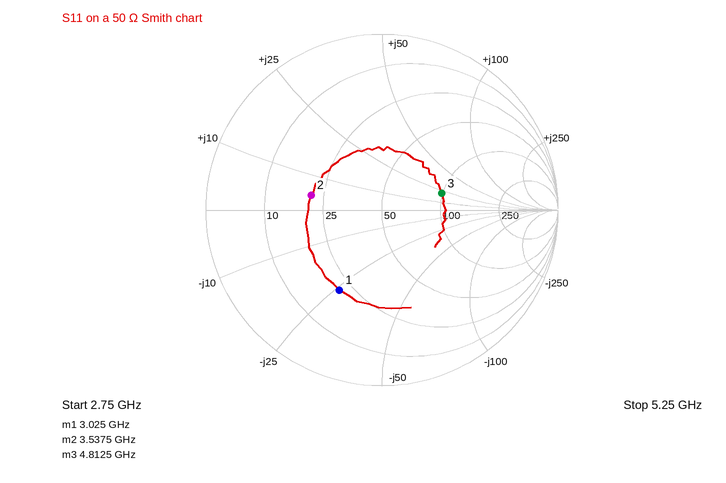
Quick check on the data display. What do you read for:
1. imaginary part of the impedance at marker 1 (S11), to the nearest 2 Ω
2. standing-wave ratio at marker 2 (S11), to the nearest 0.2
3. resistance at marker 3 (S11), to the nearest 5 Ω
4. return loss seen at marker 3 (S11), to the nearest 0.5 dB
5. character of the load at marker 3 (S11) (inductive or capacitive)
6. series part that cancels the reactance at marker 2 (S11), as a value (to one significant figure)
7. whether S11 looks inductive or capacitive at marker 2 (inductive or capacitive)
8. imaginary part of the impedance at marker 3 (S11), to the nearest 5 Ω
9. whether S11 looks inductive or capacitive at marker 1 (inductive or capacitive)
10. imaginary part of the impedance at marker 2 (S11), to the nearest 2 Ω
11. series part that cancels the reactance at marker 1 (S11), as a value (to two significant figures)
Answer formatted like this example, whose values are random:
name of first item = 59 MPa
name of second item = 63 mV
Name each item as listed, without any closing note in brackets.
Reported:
imaginary part of the impedance at marker 1 (S11), to the nearest 2 Ω = -26 Ω
standing-wave ratio at marker 2 (S11), to the nearest 0.2 = 2.4
resistance at marker 3 (S11), to the nearest 5 Ω = 100 Ω
return loss seen at marker 3 (S11), to the nearest 0.5 dB = 9.0 dB
character of the load at marker 3 (S11) = inductive
series part that cancels the reactance at marker 2 (S11), as a value = 10 pF
whether S11 looks inductive or capacitive at marker 2 = inductive
imaginary part of the impedance at marker 3 (S11), to the nearest 5 Ω = +20 Ω
whether S11 looks inductive or capacitive at marker 1 = capacitive
imaginary part of the impedance at marker 2 (S11), to the nearest 2 Ω = +4 Ω
series part that cancels the reactance at marker 1 (S11), as a value = 1.4 nH
